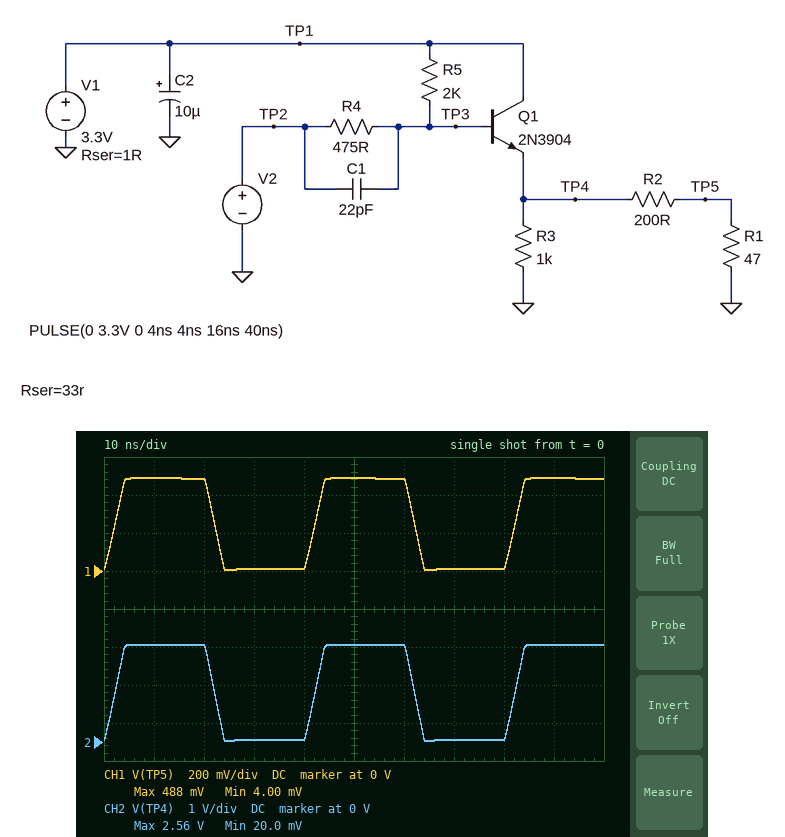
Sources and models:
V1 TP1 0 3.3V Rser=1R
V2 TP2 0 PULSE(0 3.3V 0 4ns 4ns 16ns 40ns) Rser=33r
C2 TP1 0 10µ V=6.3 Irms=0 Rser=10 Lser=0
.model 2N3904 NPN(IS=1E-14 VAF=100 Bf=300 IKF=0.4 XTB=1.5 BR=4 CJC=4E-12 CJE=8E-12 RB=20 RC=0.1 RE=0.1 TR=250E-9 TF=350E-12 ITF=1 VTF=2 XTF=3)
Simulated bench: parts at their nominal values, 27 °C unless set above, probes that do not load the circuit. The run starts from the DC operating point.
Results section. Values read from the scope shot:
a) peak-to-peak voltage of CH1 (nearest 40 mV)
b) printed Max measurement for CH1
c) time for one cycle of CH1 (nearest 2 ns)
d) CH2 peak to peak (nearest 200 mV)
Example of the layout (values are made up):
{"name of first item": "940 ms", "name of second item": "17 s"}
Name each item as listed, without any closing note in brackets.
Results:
{"peak-to-peak voltage of CH1": "480 mV", "printed Max measurement for CH1": "488 mV", "time for one cycle of CH1": "40 ns", "CH2 peak to peak": "2.6 V"}
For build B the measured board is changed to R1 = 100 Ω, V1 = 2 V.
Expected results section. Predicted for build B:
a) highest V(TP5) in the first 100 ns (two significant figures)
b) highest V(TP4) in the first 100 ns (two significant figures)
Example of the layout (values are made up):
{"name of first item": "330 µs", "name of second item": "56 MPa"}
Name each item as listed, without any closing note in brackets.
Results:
{"highest V(TP5) in the first 100 ns": "630 mV", "highest V(TP4) in the first 100 ns": "1.9 V"}
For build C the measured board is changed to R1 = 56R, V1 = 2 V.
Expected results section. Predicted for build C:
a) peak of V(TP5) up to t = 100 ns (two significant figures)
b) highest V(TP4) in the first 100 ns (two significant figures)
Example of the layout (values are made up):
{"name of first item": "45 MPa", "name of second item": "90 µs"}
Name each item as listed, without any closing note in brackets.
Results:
{"peak of V(TP5) up to t = 100 ns": "410 mV", "highest V(TP4) in the first 100 ns": "1.9 V"}
